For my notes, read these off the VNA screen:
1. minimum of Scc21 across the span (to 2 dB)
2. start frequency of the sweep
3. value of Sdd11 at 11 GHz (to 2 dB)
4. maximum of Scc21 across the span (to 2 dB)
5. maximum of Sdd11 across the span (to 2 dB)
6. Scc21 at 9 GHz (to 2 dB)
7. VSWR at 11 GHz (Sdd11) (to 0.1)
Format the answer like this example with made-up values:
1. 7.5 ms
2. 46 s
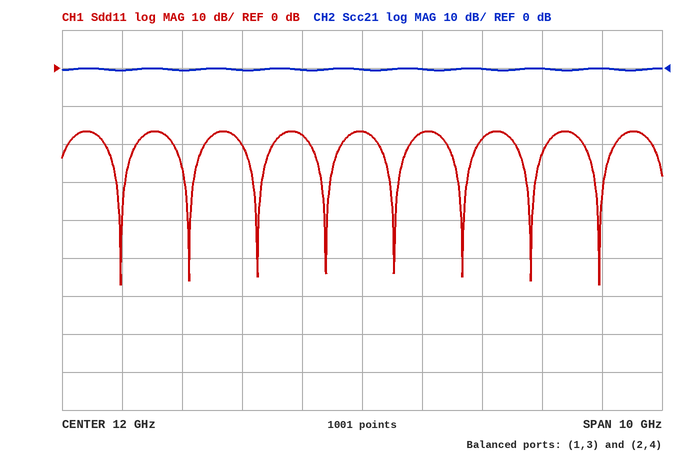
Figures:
1. 0 dB
2. 7 GHz
3. -18 dB
4. 0 dB
5. -16 dB
6. 0 dB
7. 1.3
